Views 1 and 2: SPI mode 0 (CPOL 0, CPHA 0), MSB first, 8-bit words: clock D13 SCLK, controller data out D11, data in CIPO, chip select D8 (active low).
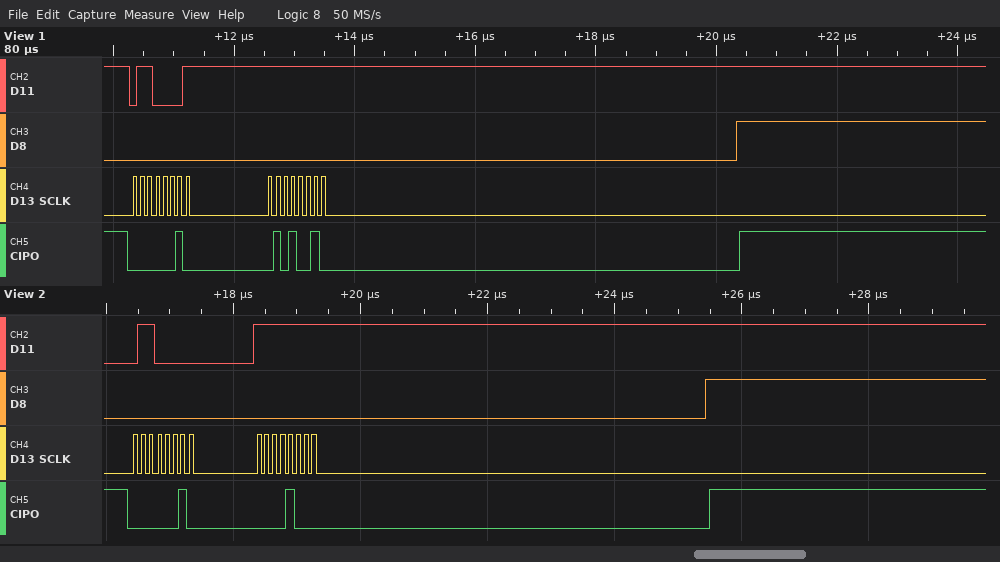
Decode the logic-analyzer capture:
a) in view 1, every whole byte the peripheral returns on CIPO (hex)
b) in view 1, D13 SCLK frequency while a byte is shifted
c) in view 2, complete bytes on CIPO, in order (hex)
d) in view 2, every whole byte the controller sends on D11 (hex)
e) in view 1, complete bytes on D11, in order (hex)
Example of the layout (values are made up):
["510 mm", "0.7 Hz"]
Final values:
["0x02 0x52", "8 MHz", "02 08", "60 FF", "0x61 0xFF"]
